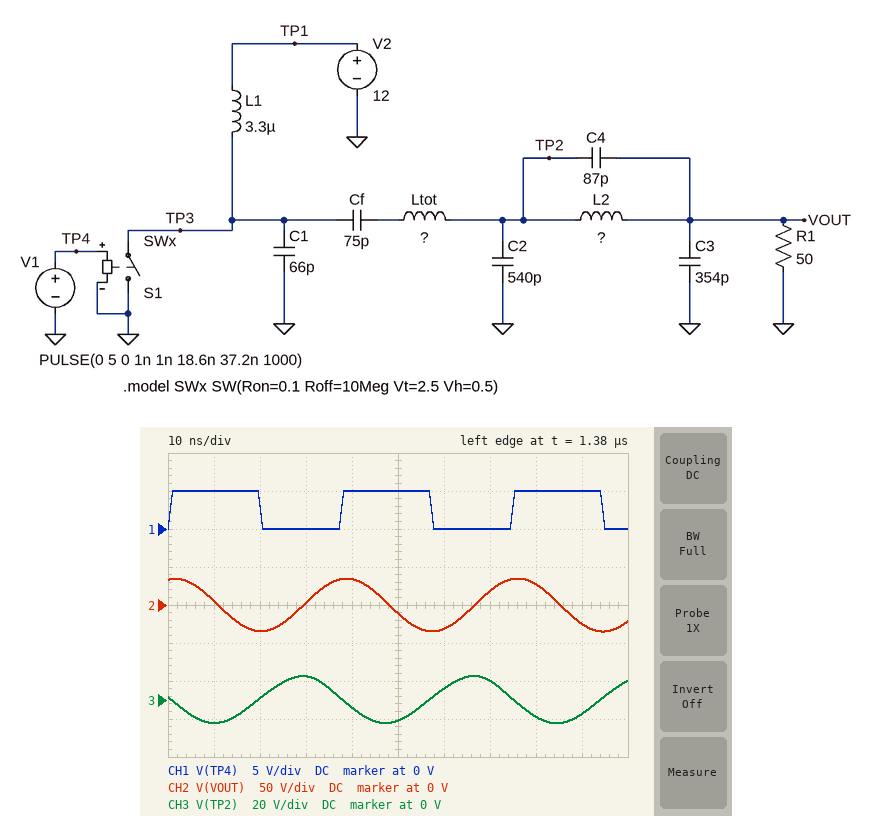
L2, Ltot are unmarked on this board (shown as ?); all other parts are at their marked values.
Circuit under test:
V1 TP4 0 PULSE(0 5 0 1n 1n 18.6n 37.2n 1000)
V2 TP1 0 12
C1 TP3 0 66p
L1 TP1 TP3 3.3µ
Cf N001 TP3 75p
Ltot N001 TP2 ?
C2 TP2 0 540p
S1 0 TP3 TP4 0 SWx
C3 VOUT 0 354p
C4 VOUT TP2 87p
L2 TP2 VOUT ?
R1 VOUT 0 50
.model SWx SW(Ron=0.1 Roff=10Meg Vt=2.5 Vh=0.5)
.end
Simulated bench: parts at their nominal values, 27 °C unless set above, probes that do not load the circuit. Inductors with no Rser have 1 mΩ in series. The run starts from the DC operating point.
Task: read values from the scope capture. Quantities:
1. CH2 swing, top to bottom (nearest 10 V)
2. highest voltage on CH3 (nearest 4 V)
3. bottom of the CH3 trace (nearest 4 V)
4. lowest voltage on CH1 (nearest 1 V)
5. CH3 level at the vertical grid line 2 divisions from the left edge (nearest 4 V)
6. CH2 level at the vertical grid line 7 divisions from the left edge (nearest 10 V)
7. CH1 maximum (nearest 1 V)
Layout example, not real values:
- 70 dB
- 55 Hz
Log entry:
- 70 V
- 12 V
- -12 V
- 0 V
- 0 V
- 20 V
- 5 V
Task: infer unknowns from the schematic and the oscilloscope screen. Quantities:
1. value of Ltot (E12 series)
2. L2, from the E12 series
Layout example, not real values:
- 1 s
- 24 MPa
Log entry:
- 470 nH
- 82 nH
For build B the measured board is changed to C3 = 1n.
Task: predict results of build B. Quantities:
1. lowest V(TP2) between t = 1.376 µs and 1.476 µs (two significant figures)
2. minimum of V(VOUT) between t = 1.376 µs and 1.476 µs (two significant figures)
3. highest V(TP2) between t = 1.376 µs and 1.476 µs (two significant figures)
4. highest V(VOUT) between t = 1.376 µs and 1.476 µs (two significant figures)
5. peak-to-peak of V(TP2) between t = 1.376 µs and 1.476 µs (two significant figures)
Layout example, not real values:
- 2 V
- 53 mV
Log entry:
- -20 V
- -9.7 V
- 19 V
- 9.8 V
- 38 V
